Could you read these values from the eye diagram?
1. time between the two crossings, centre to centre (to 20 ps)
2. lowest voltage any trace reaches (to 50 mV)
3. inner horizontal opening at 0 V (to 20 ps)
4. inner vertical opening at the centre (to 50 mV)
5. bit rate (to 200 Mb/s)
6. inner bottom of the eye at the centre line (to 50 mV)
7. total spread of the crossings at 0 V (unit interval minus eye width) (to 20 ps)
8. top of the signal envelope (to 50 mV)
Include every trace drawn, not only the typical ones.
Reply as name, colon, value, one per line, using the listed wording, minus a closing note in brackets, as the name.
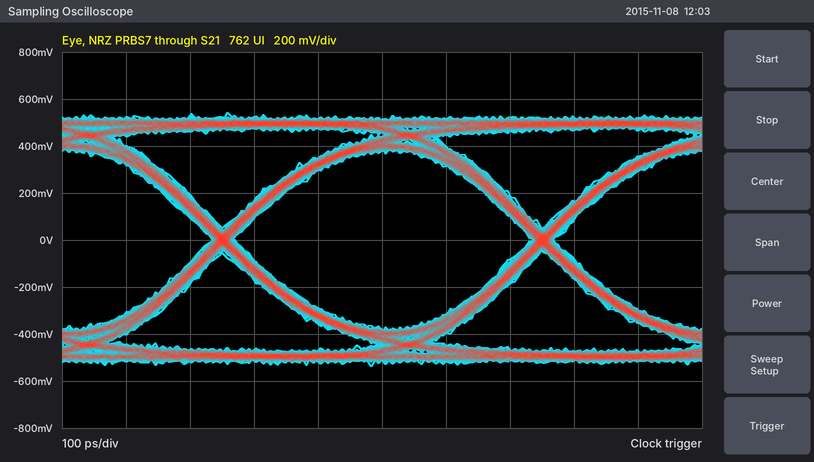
time between the two crossings, centre to centre: 500 ps
lowest voltage any trace reaches: -550 mV
inner horizontal opening at 0 V: 460 ps
inner vertical opening at the centre: 750 mV
bit rate: 2.0 Gb/s
inner bottom of the eye at the centre line: -400 mV
total spread of the crossings at 0 V (unit interval minus eye width): 40 ps
top of the signal envelope: 550 mV
